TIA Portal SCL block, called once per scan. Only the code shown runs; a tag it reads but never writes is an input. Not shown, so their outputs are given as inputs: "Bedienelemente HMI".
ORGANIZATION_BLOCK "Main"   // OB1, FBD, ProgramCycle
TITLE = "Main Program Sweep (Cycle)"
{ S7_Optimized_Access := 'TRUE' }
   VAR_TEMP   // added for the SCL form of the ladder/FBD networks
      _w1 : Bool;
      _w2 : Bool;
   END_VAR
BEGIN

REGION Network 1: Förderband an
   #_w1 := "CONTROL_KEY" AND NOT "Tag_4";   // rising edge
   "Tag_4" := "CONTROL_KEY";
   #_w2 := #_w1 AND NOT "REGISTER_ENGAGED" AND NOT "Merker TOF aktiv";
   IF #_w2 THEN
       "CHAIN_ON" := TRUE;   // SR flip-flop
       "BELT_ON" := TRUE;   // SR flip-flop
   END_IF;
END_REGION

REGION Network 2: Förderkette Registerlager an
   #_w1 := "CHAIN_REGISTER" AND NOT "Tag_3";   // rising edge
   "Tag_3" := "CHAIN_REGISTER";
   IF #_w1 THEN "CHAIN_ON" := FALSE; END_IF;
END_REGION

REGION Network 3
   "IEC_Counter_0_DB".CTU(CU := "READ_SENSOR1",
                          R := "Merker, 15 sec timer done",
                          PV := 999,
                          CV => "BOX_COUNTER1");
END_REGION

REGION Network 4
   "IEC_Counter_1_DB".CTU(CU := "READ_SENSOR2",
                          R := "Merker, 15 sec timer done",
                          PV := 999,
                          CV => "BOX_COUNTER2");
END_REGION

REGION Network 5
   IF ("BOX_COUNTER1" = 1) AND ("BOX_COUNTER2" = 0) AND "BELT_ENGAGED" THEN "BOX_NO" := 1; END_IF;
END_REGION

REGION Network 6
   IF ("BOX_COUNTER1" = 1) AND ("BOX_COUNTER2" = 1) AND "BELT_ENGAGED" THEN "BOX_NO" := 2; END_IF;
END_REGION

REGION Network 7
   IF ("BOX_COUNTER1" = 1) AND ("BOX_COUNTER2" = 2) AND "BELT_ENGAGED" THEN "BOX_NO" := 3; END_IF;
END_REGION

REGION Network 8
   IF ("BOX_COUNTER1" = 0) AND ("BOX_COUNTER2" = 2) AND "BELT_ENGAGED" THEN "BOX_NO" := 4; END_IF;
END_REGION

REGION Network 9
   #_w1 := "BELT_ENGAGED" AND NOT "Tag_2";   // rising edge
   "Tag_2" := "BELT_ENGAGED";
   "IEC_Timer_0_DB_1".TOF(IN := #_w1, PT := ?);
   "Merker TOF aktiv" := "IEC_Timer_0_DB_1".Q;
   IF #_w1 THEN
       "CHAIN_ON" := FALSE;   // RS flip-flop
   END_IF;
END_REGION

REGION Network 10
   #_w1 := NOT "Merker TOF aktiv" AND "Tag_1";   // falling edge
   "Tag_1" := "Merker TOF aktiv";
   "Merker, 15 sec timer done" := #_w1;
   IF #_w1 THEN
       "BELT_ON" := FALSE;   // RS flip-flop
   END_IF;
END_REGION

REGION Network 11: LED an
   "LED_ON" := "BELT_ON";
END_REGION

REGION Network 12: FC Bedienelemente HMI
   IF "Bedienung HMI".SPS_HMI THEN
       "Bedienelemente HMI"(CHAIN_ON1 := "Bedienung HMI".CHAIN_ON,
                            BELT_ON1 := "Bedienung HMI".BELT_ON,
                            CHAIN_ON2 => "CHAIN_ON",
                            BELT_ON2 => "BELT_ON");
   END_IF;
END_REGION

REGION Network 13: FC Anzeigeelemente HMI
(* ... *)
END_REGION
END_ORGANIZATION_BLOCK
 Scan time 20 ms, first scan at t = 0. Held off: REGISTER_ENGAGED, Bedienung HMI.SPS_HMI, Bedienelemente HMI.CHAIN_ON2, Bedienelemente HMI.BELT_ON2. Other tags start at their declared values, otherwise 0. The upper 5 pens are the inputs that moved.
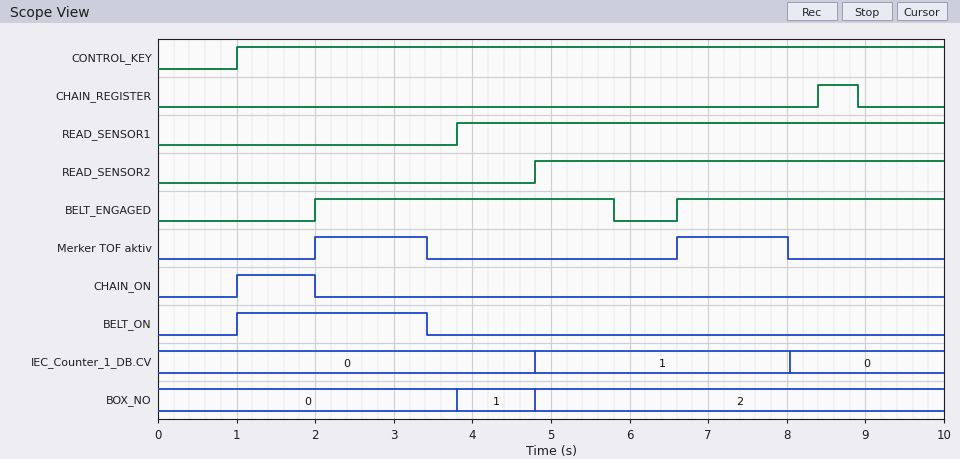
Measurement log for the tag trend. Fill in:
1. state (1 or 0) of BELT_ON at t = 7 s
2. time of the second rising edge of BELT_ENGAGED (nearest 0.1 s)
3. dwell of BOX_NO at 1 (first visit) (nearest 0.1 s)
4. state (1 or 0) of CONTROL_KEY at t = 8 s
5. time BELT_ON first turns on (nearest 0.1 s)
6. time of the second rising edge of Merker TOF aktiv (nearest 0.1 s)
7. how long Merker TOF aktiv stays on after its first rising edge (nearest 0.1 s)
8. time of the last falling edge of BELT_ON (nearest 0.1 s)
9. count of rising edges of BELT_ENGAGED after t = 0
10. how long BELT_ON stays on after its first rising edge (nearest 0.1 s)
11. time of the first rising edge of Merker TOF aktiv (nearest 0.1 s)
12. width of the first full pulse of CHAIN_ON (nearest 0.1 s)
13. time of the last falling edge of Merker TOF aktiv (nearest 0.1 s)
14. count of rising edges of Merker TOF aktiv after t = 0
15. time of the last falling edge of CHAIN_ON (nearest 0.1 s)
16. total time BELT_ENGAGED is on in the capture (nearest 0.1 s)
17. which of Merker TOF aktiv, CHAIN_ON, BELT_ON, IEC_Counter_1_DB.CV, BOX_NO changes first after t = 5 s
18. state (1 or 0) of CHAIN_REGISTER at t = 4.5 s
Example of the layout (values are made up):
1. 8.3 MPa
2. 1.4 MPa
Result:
1. 0
2. 6.6 s
3. 1.0 s
4. 1
5. 1.0 s
6. 6.6 s
7. 1.4 s
8. 3.4 s
9. 2
10. 2.4 s
11. 2.0 s
12. 1.0 s
13. 8.0 s
14. 2
15. 2.0 s
16. 7.2 s
17. Merker TOF aktiv
18. 0
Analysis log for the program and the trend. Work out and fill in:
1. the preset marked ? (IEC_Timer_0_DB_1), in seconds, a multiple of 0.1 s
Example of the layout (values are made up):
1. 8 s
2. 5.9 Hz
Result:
1. 1.4 s
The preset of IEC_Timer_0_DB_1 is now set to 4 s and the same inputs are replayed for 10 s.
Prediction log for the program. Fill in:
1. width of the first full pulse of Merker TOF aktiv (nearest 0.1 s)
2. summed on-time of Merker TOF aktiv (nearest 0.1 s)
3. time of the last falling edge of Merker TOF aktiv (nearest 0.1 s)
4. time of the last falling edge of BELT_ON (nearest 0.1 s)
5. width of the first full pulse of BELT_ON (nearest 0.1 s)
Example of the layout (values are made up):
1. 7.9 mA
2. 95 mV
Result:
1. 4.0 s
2. 7.4 s
3. 6.0 s
4. 6.0 s
5. 5.0 s
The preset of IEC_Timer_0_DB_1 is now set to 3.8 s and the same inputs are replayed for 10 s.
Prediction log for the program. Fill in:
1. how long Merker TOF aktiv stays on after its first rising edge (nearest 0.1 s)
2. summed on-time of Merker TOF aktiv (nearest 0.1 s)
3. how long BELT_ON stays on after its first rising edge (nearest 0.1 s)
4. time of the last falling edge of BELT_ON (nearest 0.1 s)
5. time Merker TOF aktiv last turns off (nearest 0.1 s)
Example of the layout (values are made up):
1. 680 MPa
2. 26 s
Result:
1. 3.8 s
2. 7.2 s
3. 4.8 s
4. 5.8 s
5. 5.8 s
